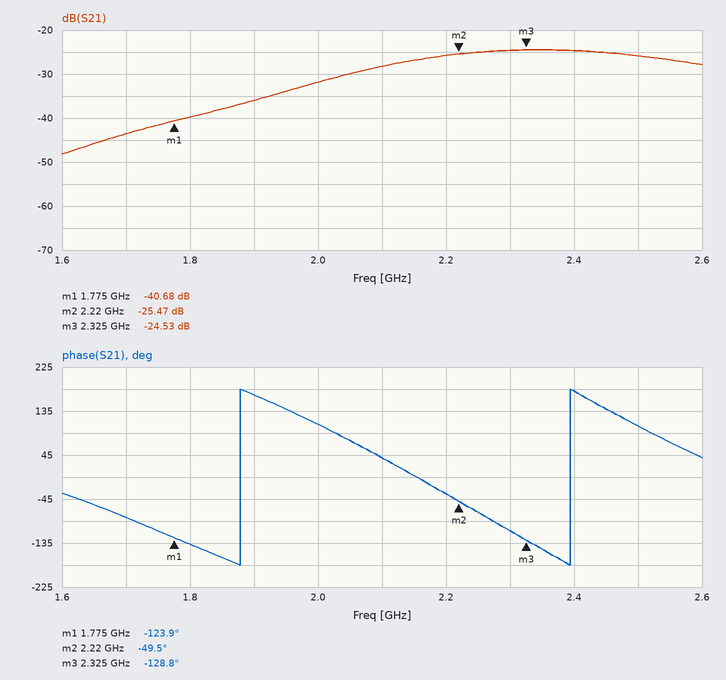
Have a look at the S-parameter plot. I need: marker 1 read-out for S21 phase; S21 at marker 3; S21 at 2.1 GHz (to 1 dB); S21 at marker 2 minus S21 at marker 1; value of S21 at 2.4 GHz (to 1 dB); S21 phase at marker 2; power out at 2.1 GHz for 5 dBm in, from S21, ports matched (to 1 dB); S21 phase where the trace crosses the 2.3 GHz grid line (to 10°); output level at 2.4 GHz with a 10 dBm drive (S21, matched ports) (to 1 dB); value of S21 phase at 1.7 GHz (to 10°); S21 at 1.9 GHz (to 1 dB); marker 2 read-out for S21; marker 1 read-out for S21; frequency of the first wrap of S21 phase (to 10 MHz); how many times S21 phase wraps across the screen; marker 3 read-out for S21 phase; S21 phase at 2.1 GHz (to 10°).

-123.9°
-24.53 dB
-28 dB
15.21 dB
-25 dB
-49.5°
-23 dBm
-110°
-15 dBm
-80°
-36 dB
-25.47 dB
-40.68 dB
1.88 GHz
2
-128.8°
40°
